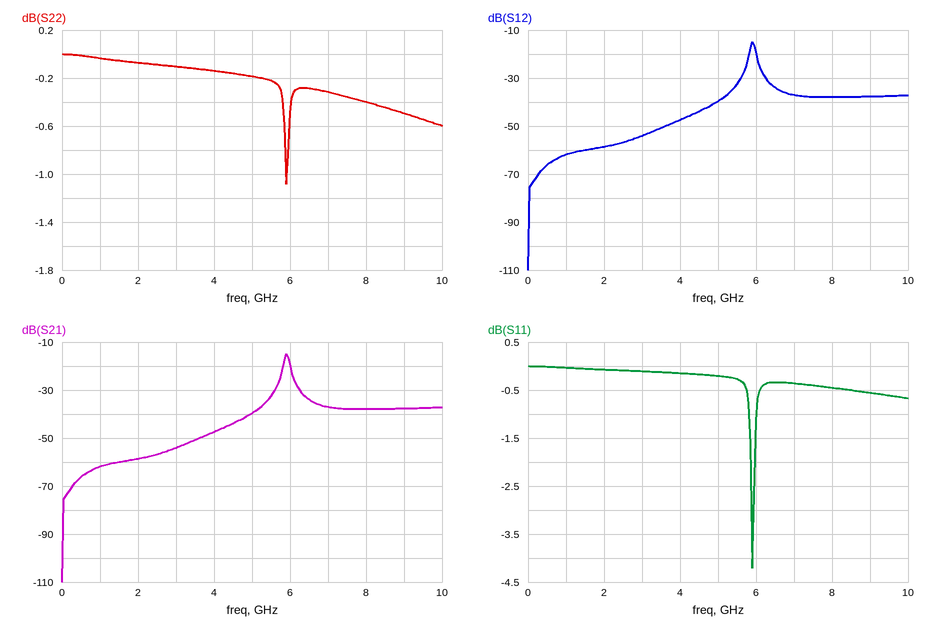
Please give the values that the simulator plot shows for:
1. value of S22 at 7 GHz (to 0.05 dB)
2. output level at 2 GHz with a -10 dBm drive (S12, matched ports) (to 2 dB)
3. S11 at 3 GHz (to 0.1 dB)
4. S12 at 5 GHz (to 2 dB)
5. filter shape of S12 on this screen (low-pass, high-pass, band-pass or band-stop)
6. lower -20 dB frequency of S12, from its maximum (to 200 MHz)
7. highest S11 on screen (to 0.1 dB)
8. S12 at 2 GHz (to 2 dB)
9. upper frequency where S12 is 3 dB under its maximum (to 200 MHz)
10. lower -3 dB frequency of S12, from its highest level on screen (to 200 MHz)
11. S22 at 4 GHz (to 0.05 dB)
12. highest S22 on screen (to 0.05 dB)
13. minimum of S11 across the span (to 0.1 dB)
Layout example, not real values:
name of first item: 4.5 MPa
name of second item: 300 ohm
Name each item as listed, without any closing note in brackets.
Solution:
value of S22 at 7 GHz: -0.30 dB
output level at 2 GHz with a -10 dBm drive (S12, matched ports): -68 dBm
S11 at 3 GHz: -0.1 dB
S12 at 5 GHz: -40 dB
filter shape of S12 on this screen: band-pass
lower -20 dB frequency of S12, from its maximum: 5.4 GHz
highest S11 on screen: 0.0 dB
S12 at 2 GHz: -58 dB
upper frequency where S12 is 3 dB under its maximum: 6.0 GHz
lower -3 dB frequency of S12, from its highest level on screen: 5.8 GHz
S22 at 4 GHz: -0.15 dB
highest S22 on screen: 0.00 dB
minimum of S11 across the span: -4.2 dB
